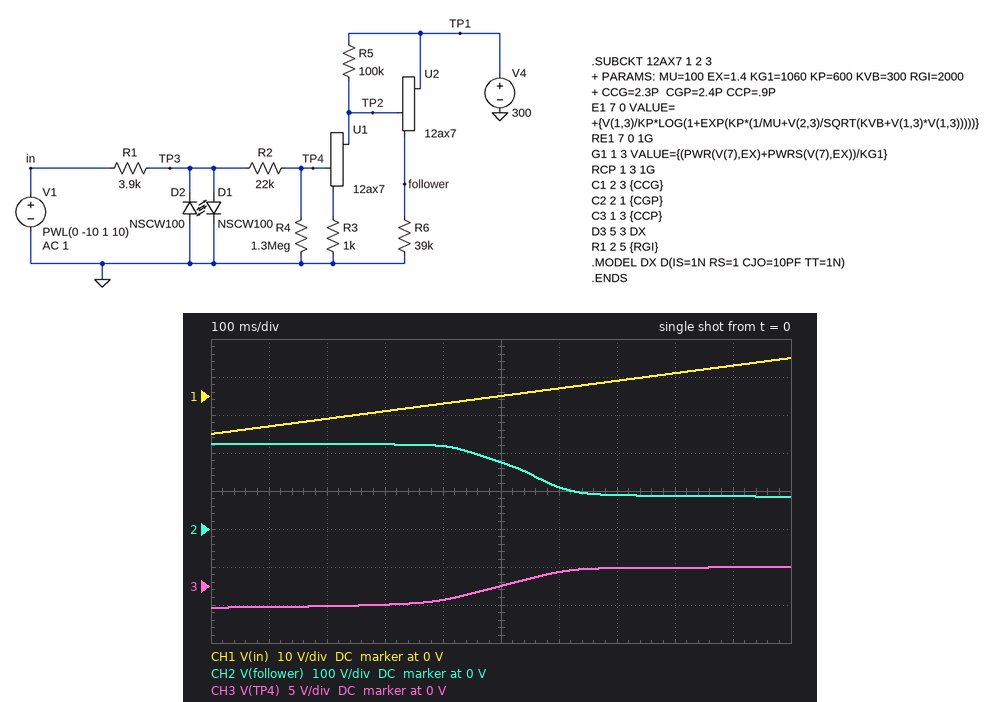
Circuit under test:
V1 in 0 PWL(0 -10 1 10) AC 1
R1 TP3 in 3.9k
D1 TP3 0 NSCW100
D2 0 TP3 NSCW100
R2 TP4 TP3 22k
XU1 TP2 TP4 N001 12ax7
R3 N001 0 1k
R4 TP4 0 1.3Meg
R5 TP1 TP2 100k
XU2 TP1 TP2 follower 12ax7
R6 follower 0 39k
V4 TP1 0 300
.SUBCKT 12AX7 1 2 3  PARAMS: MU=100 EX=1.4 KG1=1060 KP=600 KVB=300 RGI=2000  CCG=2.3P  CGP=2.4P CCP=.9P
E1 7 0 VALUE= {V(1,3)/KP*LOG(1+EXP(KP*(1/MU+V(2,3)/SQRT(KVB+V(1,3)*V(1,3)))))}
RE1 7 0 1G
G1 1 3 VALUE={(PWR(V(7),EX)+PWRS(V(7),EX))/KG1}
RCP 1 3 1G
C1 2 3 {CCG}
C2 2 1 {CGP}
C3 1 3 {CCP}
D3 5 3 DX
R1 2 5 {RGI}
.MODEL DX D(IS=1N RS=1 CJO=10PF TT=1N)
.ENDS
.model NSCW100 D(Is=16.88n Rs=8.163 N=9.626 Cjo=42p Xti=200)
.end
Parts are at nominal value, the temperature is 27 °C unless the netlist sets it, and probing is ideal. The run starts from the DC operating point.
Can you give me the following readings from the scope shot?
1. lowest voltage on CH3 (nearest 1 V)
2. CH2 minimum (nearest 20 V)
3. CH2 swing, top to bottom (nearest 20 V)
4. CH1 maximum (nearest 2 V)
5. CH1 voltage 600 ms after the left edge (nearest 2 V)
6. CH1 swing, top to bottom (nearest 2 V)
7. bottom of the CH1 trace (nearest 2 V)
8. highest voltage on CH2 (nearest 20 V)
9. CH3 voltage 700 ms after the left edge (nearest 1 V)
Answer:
-3 V
80 V
140 V
10 V
2 V
20 V
-10 V
220 V
2 V
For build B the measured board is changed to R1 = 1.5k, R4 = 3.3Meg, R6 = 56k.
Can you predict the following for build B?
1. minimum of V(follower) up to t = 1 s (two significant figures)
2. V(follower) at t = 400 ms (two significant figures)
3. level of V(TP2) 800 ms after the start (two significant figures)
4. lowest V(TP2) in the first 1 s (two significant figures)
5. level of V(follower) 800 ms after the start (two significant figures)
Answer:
83 V
230 V
84 V
82 V
85 V
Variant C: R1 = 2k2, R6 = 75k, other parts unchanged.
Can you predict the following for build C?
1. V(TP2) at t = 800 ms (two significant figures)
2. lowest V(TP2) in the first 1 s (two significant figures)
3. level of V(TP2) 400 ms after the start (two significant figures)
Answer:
85 V
83 V
240 V
